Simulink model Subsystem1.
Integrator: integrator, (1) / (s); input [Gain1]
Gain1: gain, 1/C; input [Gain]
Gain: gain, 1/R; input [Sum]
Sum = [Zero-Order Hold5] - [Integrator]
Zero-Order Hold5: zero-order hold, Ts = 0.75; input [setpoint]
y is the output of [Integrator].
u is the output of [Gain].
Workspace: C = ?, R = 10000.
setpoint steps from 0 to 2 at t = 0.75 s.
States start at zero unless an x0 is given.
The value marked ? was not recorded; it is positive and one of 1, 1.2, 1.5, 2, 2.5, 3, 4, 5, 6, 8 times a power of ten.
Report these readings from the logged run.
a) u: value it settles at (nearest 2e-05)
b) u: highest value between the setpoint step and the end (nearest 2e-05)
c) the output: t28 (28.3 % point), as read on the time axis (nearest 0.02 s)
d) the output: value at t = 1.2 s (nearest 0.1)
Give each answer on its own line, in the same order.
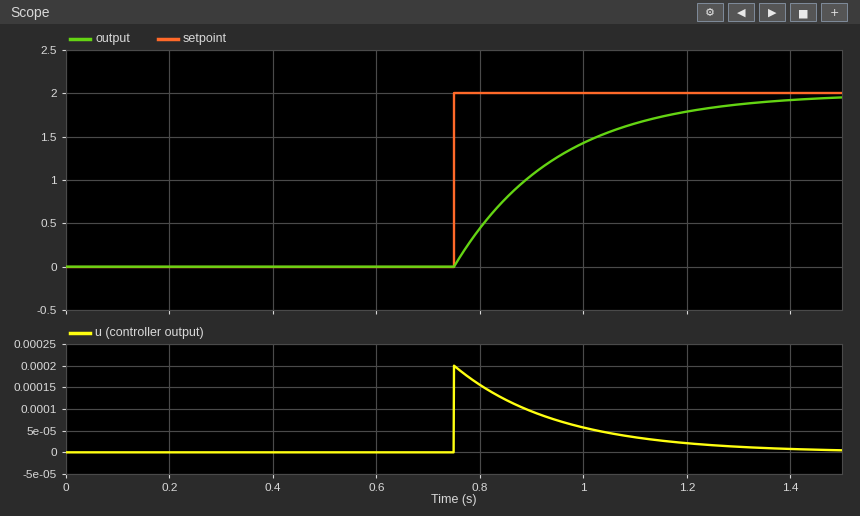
0.00000
0.00020
0.82 s
1.8
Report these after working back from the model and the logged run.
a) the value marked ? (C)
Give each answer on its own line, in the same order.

2e-05
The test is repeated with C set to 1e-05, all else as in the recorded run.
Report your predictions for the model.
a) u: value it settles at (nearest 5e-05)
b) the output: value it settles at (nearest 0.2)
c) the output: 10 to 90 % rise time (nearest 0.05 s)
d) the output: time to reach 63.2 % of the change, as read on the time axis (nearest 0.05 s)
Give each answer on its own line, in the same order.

0.00000
2.0
0.20 s
0.85 s
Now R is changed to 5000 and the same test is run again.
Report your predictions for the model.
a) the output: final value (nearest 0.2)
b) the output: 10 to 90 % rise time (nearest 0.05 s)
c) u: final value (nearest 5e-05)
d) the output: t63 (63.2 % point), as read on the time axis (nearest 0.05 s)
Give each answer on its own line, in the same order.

2.0
0.20 s
0.00000
0.85 s
